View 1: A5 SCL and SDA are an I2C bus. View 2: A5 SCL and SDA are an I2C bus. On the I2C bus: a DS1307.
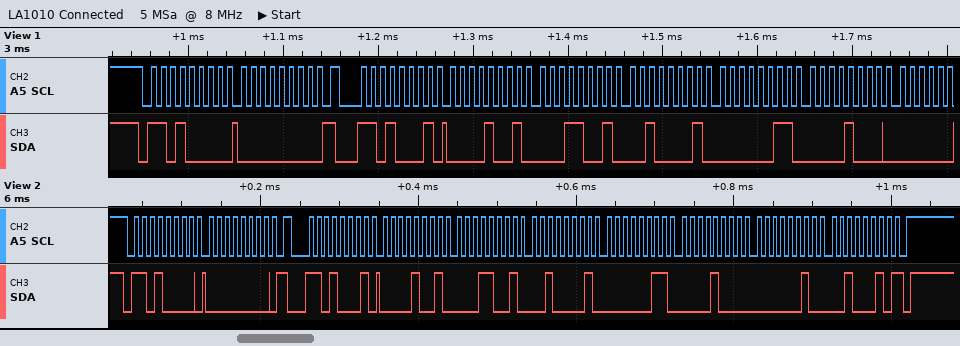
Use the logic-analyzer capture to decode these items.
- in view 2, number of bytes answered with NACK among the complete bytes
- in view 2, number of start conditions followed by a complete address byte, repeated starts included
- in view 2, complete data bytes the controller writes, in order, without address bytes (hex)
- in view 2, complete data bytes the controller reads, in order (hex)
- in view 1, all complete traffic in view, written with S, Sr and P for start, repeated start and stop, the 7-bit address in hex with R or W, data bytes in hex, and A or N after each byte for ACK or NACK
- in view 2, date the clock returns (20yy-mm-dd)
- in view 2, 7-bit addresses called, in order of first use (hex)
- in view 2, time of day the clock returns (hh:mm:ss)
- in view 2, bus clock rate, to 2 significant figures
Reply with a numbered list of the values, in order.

1. 1
2. 2
3. 00
4. 09 19 21 03 08 02 22
5. S 68W A 00 A Sr 68R A 09 A 19 A 21 A 03 A 08 A
6. 2022-02-08
7. 0x68
8. 21:19:09
9. 100 kHz
